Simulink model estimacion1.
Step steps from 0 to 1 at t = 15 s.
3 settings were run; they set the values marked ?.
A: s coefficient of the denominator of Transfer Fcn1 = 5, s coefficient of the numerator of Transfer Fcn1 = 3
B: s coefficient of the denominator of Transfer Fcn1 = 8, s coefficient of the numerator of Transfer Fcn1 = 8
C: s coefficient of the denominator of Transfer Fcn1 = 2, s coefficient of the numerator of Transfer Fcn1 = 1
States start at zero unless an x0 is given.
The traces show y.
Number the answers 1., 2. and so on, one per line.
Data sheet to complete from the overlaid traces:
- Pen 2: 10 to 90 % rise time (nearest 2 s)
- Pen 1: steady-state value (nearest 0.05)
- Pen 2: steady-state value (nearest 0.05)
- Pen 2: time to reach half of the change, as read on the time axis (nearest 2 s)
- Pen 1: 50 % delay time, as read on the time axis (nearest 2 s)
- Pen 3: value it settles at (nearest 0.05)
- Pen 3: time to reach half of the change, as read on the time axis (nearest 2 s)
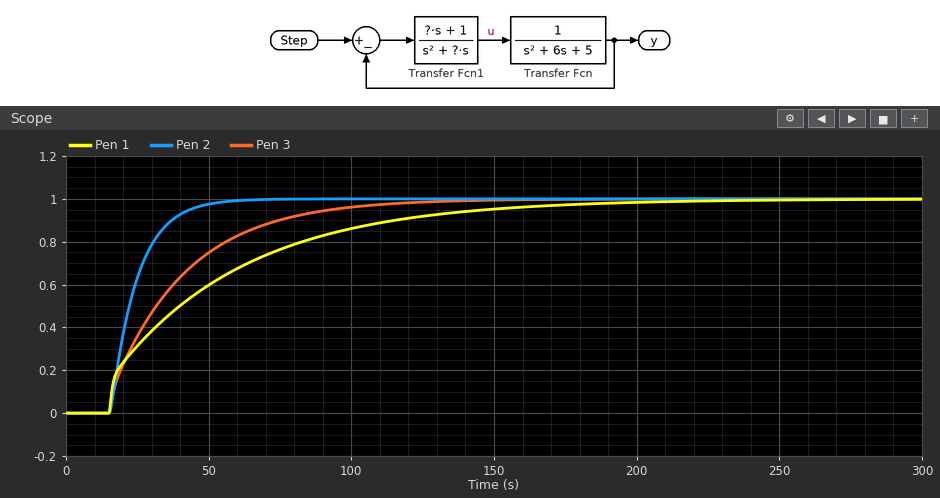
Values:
1. 20 s
2. 1.00
3. 1.00
4. 22 s
5. 40 s
6. 1.00
7. 32 s
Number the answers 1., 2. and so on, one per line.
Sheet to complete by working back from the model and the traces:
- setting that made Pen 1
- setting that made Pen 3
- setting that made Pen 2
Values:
1. B
2. A
3. C
